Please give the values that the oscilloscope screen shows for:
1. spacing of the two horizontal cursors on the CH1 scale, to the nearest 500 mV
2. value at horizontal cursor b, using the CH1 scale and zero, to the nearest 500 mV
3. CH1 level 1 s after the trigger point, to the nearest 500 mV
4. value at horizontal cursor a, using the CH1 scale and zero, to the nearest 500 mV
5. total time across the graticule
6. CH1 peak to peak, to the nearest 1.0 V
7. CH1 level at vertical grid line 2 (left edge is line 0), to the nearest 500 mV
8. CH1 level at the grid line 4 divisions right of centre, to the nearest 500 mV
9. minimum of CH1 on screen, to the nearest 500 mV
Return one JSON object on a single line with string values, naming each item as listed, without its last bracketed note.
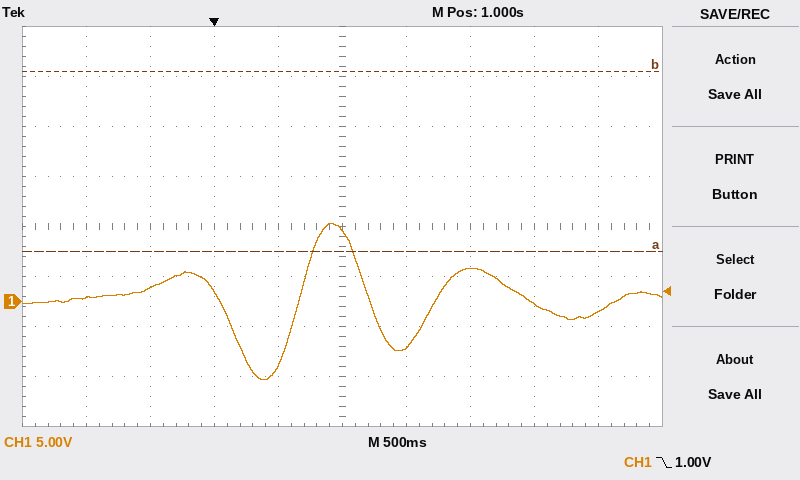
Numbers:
{"spacing of the two horizontal cursors on the CH1 scale, to the nearest 500 mV": "18.0 V", "value at horizontal cursor b, using the CH1 scale and zero, to the nearest 500 mV": "23.0 V", "CH1 level 1 s after the trigger point, to the nearest 500 mV": "7.0 V", "value at horizontal cursor a, using the CH1 scale and zero, to the nearest 500 mV": "5.0 V", "total time across the graticule": "5 s", "CH1 peak to peak, to the nearest 1.0 V": "16.0 V", "CH1 level at vertical grid line 2 (left edge is line 0), to the nearest 500 mV": "1.5 V", "CH1 level at the grid line 4 divisions right of centre, to the nearest 500 mV": "-1.0 V", "minimum of CH1 on screen, to the nearest 500 mV": "-8.0 V"}
